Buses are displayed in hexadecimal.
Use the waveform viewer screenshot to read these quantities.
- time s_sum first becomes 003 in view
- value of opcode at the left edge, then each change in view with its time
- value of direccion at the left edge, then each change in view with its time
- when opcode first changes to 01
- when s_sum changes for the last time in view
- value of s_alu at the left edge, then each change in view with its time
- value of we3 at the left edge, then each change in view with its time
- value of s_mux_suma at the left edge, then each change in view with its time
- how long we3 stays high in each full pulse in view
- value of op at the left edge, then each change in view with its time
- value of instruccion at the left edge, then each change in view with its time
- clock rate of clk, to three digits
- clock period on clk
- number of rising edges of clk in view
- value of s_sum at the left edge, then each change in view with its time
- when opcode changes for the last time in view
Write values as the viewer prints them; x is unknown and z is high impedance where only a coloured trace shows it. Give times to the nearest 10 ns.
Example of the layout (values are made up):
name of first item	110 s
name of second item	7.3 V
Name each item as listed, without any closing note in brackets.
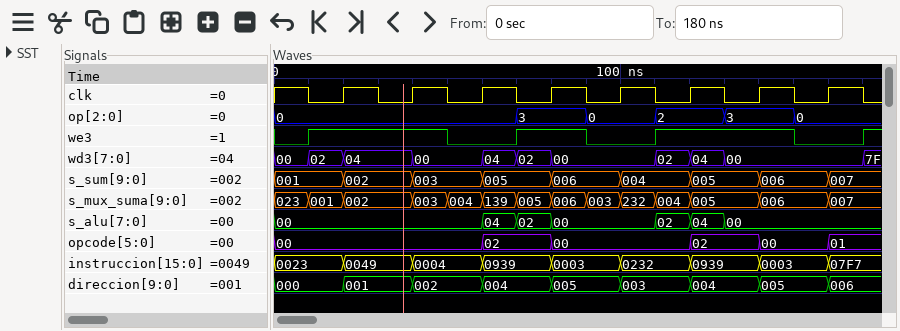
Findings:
time s_sum first becomes 003 in view	40 ns
value of opcode at the left edge, then each change in view with its time	00, 02 at 60 ns, 00 at 80 ns, 02 at 120 ns, 00 at 140 ns, 01 at 160 ns
value of direccion at the left edge, then each change in view with its time	000, 001 at 20 ns, 002 at 40 ns, 004 at 60 ns, 005 at 80 ns, 003 at 100 ns, 004 at 120 ns, 005 at 140 ns, 006 at 160 ns
when opcode first changes to 01	160 ns
when s_sum changes for the last time in view	160 ns
value of s_alu at the left edge, then each change in view with its time	00, 04 at 60 ns, 02 at 70 ns, 00 at 80 ns, 02 at 110 ns, 04 at 120 ns, 00 at 130 ns
value of we3 at the left edge, then each change in view with its time	0, 1 at 10 ns, 0 at 50 ns, 1 at 70 ns, 0 at 90 ns, 1 at 110 ns, 0 at 150 ns, 1 at 170 ns
value of s_mux_suma at the left edge, then each change in view with its time	023, 001 at 10 ns, 002 at 20 ns, 003 at 40 ns, 004 at 50 ns, 139 at 60 ns, 005 at 70 ns, 006 at 80 ns, 003 at 90 ns, 232 at 100 ns, 004 at 110 ns, 005 at 120 ns, 006 at 140 ns, 007 at 160 ns
how long we3 stays high in each full pulse in view	40 ns, 20 ns, 40 ns
value of op at the left edge, then each change in view with its time	0, 3 at 70 ns, 0 at 90 ns, 2 at 110 ns, 3 at 130 ns, 0 at 150 ns
value of instruccion at the left edge, then each change in view with its time	0023, 0049 at 20 ns, 0004 at 40 ns, 0939 at 60 ns, 0003 at 80 ns, 0232 at 100 ns, 0939 at 120 ns, 0003 at 140 ns, 07F7 at 160 ns
clock rate of clk, to three digits	50.0 MHz
clock period on clk	20 ns
number of rising edges of clk in view	8
value of s_sum at the left edge, then each change in view with its time	001, 002 at 20 ns, 003 at 40 ns, 005 at 60 ns, 006 at 80 ns, 004 at 100 ns, 005 at 120 ns, 006 at 140 ns, 007 at 160 ns
when opcode changes for the last time in view	160 ns
